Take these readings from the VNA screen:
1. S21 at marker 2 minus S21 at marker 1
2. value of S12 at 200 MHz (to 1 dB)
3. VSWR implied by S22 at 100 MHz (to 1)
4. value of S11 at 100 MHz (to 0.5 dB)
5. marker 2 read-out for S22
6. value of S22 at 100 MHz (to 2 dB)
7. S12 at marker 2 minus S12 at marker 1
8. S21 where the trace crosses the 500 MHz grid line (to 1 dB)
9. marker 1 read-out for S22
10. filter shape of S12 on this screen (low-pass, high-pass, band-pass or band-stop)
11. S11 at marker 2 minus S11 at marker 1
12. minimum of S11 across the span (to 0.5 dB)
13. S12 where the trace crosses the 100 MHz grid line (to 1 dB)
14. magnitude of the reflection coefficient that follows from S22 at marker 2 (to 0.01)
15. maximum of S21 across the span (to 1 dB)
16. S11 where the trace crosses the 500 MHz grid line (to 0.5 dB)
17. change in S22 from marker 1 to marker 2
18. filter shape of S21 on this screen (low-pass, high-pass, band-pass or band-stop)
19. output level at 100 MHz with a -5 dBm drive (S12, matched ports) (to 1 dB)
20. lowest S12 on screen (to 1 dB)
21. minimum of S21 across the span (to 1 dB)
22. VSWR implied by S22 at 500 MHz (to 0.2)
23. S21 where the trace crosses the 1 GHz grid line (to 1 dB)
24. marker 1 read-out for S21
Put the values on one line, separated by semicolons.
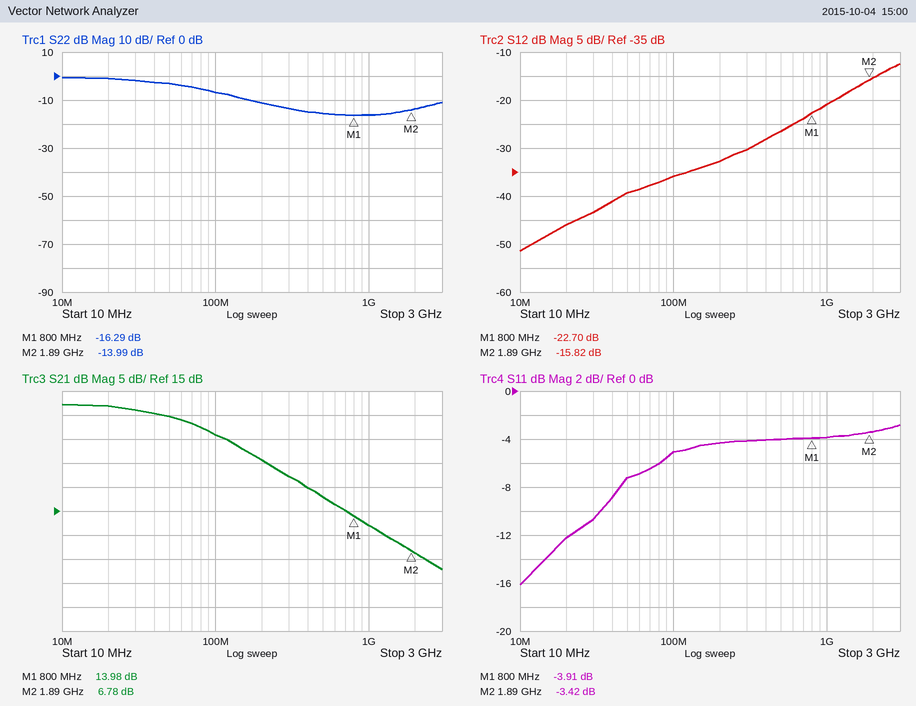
-7.20 dB; -33 dB; 3; -5.0 dB; -13.99 dB; -6 dB; 6.88 dB; 18 dB; -16.29 dB; high-pass; 0.49 dB; -16.0 dB; -36 dB; 0.20; 37 dB; -4.0 dB; 2.30 dB; low-pass; -41 dBm; -51 dB; 3 dB; 1.4; 12 dB; 13.98 dB
